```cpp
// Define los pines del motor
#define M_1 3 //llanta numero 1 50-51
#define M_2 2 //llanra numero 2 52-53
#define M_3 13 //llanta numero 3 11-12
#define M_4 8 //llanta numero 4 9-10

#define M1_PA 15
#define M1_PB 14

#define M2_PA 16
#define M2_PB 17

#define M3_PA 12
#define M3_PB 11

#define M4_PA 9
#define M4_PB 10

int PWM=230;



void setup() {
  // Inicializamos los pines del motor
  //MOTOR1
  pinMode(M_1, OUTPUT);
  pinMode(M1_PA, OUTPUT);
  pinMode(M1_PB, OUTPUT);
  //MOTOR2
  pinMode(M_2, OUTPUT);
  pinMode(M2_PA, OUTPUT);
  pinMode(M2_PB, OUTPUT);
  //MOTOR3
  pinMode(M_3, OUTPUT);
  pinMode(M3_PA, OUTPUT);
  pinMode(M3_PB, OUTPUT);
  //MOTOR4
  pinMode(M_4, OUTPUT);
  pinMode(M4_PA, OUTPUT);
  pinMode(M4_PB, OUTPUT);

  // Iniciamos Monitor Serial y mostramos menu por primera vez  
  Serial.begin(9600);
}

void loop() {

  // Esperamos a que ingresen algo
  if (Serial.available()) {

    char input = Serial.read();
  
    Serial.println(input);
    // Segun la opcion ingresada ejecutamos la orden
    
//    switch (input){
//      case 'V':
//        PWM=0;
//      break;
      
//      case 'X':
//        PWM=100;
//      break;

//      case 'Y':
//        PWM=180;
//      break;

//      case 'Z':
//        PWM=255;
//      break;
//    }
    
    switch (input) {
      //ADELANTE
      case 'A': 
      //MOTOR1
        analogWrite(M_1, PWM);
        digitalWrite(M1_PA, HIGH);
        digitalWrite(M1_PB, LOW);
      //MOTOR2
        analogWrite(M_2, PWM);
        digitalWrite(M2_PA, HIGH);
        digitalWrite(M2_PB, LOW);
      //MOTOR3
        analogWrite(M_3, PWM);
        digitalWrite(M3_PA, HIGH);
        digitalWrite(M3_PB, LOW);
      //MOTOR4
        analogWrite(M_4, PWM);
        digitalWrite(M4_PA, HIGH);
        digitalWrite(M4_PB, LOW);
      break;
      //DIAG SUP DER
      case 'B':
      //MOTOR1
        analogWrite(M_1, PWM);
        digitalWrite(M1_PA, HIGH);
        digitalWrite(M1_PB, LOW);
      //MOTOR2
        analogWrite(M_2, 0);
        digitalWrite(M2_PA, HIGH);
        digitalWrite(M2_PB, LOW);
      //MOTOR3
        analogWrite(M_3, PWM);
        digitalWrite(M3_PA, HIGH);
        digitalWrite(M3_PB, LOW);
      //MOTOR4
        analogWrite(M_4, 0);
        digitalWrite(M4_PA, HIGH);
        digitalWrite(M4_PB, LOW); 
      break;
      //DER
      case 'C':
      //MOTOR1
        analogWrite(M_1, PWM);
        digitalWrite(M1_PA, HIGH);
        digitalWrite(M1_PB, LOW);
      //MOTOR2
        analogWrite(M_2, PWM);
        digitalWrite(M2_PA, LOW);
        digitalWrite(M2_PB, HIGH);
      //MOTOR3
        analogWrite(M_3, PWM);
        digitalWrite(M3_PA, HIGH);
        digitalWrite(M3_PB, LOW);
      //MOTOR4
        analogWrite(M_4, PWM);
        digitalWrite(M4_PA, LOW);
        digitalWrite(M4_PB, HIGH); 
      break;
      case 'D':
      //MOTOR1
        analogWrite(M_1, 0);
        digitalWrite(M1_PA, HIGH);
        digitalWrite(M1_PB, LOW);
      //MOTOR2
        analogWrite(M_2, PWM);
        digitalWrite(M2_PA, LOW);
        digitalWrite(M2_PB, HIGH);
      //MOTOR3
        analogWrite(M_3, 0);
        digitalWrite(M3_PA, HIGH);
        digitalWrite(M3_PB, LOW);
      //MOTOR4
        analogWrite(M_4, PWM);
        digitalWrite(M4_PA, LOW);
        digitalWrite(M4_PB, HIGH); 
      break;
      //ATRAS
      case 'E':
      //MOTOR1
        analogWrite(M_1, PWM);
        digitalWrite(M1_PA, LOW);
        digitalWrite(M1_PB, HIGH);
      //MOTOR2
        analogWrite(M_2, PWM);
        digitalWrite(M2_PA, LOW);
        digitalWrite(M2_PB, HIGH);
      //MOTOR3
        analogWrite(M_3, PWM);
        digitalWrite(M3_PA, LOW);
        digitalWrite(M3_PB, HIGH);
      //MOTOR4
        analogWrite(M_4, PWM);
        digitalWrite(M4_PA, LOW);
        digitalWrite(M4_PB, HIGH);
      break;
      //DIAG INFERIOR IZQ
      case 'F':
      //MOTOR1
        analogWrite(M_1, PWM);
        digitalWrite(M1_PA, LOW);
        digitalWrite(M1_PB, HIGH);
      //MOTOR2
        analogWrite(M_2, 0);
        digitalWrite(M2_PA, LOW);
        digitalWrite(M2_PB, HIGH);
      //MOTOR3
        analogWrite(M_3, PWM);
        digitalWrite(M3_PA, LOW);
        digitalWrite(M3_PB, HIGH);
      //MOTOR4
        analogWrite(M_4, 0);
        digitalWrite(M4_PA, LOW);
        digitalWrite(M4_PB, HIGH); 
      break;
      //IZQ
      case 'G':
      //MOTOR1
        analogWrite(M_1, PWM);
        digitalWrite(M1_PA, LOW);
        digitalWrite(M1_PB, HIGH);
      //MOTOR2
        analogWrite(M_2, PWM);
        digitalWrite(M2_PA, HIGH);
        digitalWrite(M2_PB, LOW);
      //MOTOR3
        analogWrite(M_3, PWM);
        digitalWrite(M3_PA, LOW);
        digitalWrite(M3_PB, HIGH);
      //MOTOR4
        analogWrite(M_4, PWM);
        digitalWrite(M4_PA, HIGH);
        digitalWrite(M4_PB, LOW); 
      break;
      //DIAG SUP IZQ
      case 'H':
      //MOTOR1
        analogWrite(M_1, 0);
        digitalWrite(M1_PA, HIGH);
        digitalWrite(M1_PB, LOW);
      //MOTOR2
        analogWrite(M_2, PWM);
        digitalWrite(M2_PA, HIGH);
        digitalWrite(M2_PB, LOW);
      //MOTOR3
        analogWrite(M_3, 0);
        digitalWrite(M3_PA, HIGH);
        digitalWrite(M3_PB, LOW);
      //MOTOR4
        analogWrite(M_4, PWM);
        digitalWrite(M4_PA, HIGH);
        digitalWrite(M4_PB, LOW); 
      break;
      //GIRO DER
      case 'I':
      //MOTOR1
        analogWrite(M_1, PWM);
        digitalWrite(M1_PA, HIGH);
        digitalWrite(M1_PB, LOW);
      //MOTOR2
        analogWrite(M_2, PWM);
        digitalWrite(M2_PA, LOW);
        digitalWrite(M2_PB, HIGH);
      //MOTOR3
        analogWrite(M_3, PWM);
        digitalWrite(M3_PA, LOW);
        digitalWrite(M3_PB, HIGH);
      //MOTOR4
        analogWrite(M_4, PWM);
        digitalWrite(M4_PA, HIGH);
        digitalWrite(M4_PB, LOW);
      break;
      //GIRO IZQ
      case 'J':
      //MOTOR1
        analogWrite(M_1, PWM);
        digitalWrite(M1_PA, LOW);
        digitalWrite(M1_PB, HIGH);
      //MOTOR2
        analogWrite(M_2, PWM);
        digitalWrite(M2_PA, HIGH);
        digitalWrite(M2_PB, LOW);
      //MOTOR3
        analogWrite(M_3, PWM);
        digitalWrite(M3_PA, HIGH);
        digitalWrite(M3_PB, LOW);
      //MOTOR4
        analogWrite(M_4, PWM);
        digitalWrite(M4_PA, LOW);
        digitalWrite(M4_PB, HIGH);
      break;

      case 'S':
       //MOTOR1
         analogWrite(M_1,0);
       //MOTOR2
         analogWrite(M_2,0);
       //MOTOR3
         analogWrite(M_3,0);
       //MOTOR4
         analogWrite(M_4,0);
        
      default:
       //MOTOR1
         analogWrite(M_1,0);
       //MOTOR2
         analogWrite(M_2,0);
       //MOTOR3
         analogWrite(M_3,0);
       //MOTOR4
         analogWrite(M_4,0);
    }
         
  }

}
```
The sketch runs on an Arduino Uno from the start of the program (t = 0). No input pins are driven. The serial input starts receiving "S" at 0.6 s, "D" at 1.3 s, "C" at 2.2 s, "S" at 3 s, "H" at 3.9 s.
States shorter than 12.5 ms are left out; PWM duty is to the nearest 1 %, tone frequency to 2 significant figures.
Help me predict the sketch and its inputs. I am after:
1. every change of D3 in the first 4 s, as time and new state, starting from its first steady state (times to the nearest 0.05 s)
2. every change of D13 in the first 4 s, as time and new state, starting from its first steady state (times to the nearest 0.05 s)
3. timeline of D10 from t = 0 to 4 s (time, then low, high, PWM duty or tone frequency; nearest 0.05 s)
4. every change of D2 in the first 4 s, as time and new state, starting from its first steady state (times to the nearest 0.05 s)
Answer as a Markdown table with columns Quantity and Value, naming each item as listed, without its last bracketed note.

| Quantity | Value |
|---|---|
| every change of D3 in the first 4 s, as time and new state, starting from its first steady state | 0 s low; 2.2 s PWM 90 %; 3 s low |
| every change of D13 in the first 4 s, as time and new state, starting from its first steady state | 0 s low; 2.2 s high; 3 s low |
| timeline of D10 from t = 0 to 4 s | 0 s low; 1.3 s high; 3.9 s low |
| every change of D2 in the first 4 s, as time and new state, starting from its first steady state | 0 s low; 1.3 s high; 3 s low; 3.9 s high |
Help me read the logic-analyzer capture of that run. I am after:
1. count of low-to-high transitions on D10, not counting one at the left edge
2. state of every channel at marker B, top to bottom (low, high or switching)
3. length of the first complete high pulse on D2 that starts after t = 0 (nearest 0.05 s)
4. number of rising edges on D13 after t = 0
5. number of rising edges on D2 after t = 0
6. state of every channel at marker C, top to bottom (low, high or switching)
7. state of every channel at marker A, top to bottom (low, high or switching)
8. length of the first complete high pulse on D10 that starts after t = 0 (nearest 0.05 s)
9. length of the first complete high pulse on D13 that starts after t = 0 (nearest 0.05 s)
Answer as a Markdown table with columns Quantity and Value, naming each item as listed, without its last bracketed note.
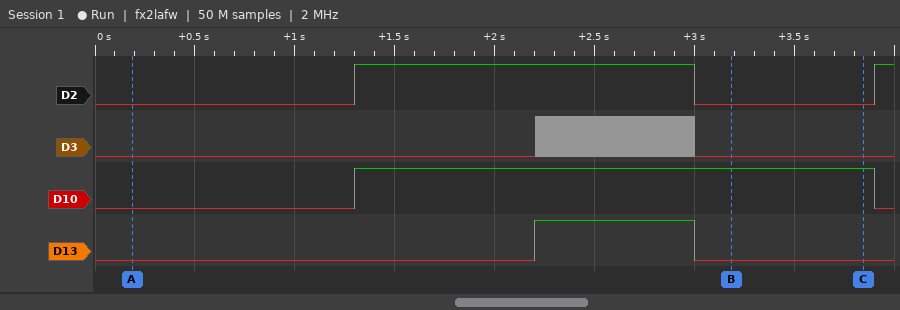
| Quantity | Value |
|---|---|
| count of low-to-high transitions on D10, not counting one at the left edge | 1 |
| state of every channel at marker B, top to bottom | D2 low, D3 low, D10 high, D13 low |
| length of the first complete high pulse on D2 that starts after t = 0 | 1.70 s |
| number of rising edges on D13 after t = 0 | 1 |
| number of rising edges on D2 after t = 0 | 2 |
| state of every channel at marker C, top to bottom | D2 low, D3 low, D10 high, D13 low |
| state of every channel at marker A, top to bottom | D2 low, D3 low, D10 low, D13 low |
| length of the first complete high pulse on D10 that starts after t = 0 | 2.60 s |
| length of the first complete high pulse on D13 that starts after t = 0 | 0.80 s |
